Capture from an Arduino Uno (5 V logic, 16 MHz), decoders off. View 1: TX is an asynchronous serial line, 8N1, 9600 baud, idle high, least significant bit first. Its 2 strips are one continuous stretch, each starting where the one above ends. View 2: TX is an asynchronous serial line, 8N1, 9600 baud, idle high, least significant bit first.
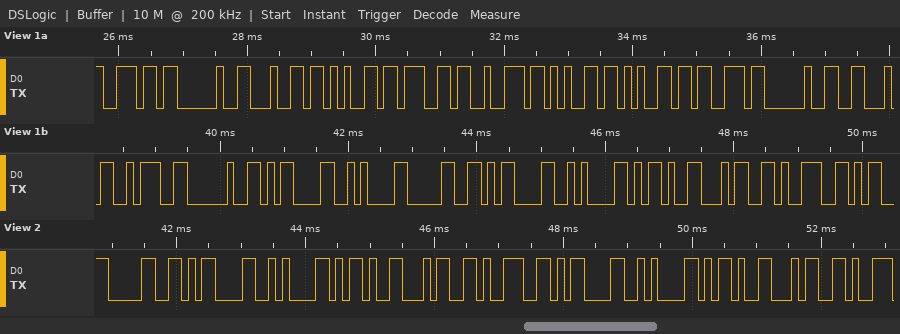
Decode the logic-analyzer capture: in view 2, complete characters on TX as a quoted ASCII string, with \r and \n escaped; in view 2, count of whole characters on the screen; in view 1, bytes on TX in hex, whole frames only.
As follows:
"0\r\n-49\r\n-4"
10
0x6E 0x20 0x64 0x65 0x67 0x72 0x65 0x65 0x73 0x20 0x46 0x3A 0x20 0x0D 0x0A 0x30 0x0D 0x0A 0x2D 0x34 0x39
